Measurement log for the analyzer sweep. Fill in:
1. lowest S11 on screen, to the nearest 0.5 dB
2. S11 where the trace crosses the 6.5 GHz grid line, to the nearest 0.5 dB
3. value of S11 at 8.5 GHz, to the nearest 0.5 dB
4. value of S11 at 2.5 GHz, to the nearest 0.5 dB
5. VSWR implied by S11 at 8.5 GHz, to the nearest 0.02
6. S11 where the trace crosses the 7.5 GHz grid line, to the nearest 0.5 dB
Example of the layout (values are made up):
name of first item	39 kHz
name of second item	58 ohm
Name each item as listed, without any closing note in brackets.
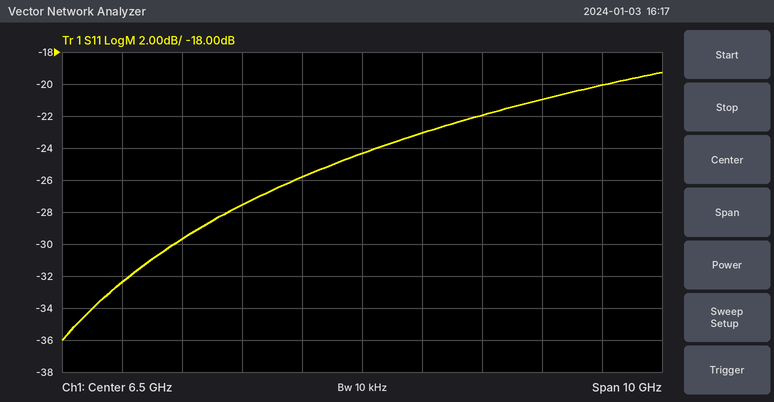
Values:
lowest S11 on screen, to the nearest 0.5 dB	-36.0 dB
S11 where the trace crosses the 6.5 GHz grid line, to the nearest 0.5 dB	-24.5 dB
value of S11 at 8.5 GHz, to the nearest 0.5 dB	-22.0 dB
value of S11 at 2.5 GHz, to the nearest 0.5 dB	-32.5 dB
VSWR implied by S11 at 8.5 GHz, to the nearest 0.02	1.18
S11 where the trace crosses the 7.5 GHz grid line, to the nearest 0.5 dB	-23.0 dB
